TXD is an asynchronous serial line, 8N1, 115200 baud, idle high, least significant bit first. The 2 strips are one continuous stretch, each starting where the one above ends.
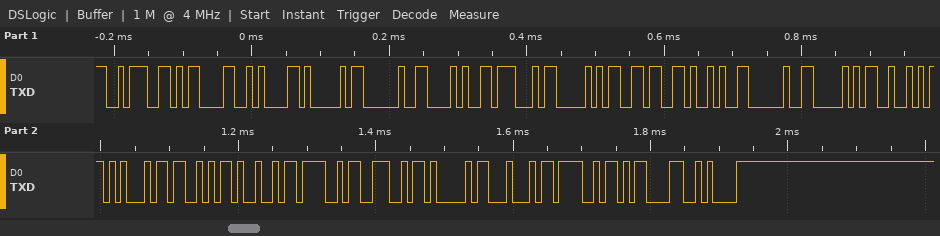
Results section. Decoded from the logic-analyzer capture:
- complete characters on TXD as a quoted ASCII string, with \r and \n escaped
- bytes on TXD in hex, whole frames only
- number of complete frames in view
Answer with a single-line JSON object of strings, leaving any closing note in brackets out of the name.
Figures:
{"complete characters on TXD as a quoted ASCII string, with \\r and \\n escaped": "\":\\r\\nA (GP6) PRESIONADO\\r\\n\"", "bytes on TXD in hex, whole frames only": "0x3A 0x0D 0x0A 0x41 0x20 0x28 0x47 0x50 0x36 0x29 0x20 0x50 0x52 0x45 0x53 0x49 0x4F 0x4E 0x41 0x44 0x4F 0x0D 0x0A", "number of complete frames in view": "23"}
